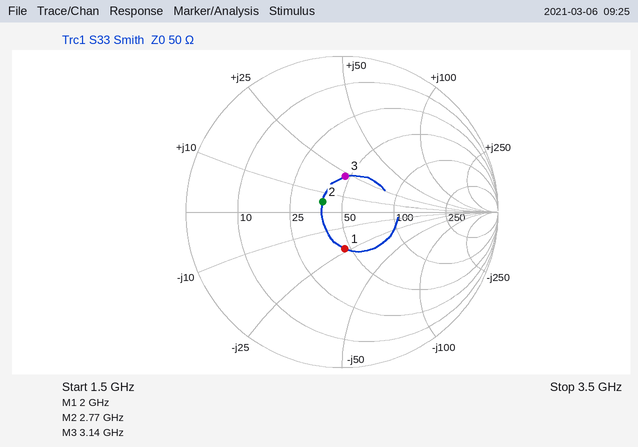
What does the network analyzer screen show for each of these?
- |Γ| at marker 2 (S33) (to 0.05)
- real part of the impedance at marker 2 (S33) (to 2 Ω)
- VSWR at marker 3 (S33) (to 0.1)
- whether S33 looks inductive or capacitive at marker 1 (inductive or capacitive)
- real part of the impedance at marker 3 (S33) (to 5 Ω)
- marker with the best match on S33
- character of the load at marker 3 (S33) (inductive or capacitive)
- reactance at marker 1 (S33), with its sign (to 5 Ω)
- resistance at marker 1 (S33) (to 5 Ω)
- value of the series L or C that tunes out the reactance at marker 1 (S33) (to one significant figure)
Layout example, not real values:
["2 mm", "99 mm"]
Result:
["0.15", "38 Ω", "1.6", "capacitive", "45 Ω", "marker 2", "inductive", "-25 Ω", "45 Ω", "2 nH"]
